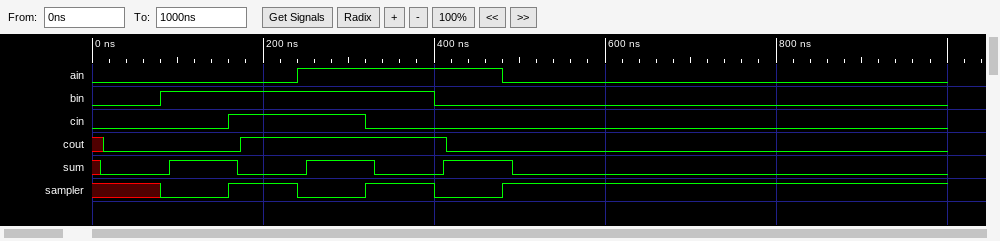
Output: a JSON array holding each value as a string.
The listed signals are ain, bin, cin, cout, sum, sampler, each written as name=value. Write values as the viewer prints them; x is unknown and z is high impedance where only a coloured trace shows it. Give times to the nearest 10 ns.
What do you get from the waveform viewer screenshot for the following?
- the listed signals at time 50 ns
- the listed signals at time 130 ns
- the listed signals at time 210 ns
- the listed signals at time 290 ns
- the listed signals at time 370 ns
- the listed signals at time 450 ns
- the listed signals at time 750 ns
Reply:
["ain=0, bin=0, cin=0, cout=0, sum=0, sampler=x", "ain=0, bin=1, cin=0, cout=0, sum=1, sampler=0", "ain=0, bin=1, cin=1, cout=1, sum=0, sampler=1", "ain=1, bin=1, cin=1, cout=1, sum=1, sampler=0", "ain=1, bin=1, cin=0, cout=1, sum=0, sampler=1", "ain=1, bin=0, cin=0, cout=0, sum=1, sampler=0", "ain=0, bin=0, cin=0, cout=0, sum=0, sampler=1"]
